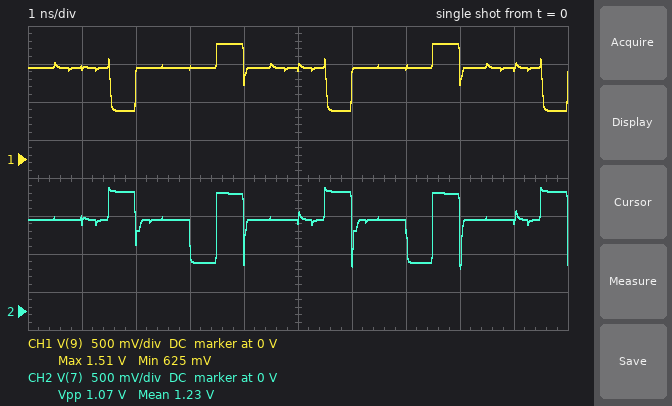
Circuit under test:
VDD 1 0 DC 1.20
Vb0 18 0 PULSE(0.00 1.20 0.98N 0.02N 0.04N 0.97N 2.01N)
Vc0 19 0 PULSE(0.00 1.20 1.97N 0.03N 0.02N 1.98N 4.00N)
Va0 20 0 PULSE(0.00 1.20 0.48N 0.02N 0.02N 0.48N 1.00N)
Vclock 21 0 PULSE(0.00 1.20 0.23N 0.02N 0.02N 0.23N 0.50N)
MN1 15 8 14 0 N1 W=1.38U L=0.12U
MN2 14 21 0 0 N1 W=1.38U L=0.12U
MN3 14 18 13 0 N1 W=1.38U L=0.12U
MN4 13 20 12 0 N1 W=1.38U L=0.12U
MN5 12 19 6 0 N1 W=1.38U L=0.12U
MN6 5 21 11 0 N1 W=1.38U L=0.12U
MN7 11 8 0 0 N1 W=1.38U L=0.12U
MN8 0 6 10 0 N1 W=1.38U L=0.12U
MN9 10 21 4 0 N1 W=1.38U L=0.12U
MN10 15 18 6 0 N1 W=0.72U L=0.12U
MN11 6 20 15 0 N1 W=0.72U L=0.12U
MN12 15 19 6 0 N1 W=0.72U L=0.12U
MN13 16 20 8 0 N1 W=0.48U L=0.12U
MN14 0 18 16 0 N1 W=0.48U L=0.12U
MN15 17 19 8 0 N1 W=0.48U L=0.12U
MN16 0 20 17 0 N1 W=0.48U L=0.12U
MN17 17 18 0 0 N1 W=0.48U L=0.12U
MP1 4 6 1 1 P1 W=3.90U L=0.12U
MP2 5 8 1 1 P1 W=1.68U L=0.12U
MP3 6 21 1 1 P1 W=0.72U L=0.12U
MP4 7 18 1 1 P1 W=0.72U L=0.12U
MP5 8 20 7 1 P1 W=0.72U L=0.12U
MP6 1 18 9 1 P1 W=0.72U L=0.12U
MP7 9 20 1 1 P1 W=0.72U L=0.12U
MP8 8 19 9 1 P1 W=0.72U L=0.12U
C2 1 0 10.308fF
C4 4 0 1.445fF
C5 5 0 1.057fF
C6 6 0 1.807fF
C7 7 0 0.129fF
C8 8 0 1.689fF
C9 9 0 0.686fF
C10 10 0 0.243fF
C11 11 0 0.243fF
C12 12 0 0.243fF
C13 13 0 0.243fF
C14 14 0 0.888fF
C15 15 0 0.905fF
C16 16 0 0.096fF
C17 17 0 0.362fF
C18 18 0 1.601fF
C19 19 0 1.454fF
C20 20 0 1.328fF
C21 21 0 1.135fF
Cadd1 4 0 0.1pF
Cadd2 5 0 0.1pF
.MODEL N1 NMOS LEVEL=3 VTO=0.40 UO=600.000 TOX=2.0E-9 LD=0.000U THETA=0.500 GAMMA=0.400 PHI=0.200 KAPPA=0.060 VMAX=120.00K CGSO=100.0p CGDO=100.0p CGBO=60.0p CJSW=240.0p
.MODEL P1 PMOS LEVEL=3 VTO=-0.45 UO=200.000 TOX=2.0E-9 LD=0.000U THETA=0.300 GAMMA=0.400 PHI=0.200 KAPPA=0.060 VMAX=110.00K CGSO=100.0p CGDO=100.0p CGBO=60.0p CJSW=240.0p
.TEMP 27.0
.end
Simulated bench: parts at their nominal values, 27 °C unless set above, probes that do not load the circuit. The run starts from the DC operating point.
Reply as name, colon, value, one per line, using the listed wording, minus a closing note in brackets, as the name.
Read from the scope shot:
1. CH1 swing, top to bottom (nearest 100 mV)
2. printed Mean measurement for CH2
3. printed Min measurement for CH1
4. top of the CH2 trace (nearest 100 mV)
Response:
CH1 swing, top to bottom: 900 mV
printed Mean measurement for CH2: 1.23 V
printed Min measurement for CH1: 625 mV
top of the CH2 trace: 1.6 V
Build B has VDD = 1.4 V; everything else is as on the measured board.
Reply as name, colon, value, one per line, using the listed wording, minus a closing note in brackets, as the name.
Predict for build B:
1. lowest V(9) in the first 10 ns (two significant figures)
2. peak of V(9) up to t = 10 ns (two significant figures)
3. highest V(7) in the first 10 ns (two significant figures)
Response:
lowest V(9) in the first 10 ns: 660 mV
peak of V(9) up to t = 10 ns: 1.6 V
highest V(7) in the first 10 ns: 1.7 V
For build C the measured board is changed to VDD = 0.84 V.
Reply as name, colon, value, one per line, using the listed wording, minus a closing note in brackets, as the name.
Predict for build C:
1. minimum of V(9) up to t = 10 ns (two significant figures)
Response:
minimum of V(9) up to t = 10 ns: 550 mV
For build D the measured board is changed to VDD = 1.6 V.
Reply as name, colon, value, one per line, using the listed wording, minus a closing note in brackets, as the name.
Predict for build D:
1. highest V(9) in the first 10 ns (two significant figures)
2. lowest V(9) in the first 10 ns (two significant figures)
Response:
highest V(9) in the first 10 ns: 1.7 V
lowest V(9) in the first 10 ns: 700 mV
